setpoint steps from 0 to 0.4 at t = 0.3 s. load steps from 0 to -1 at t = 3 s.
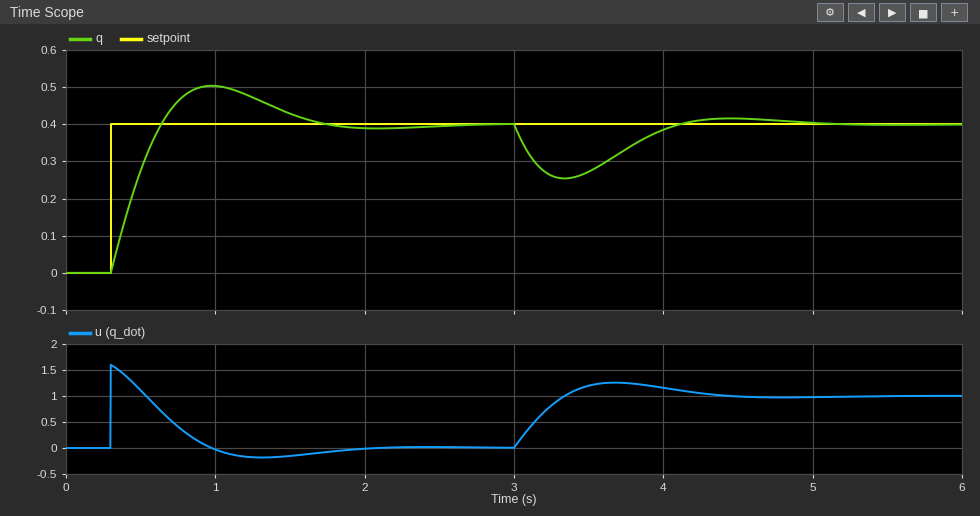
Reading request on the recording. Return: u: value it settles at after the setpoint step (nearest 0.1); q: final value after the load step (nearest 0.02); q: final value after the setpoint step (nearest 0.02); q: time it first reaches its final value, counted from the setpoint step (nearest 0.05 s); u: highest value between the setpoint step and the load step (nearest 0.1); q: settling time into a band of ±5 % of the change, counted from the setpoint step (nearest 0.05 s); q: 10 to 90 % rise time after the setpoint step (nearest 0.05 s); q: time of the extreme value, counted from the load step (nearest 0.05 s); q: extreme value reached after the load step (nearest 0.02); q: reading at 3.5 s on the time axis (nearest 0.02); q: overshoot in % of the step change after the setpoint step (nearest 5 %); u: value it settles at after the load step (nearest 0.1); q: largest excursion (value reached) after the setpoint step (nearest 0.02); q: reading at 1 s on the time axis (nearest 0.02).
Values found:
0.0
0.40
0.40
0.35 s
1.6
1.25 s
0.25 s
0.35 s
0.26
0.28
25 %
1.0
0.50
0.50
